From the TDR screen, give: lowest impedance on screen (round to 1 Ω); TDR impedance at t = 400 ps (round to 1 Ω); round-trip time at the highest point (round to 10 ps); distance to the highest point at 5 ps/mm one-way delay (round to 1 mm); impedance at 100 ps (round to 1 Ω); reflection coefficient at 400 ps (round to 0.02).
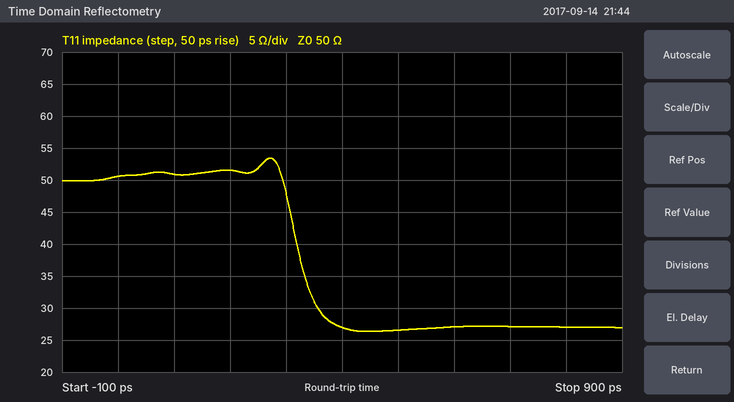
26 Ω
27 Ω
270 ps
27 mm
51 Ω
-0.30
